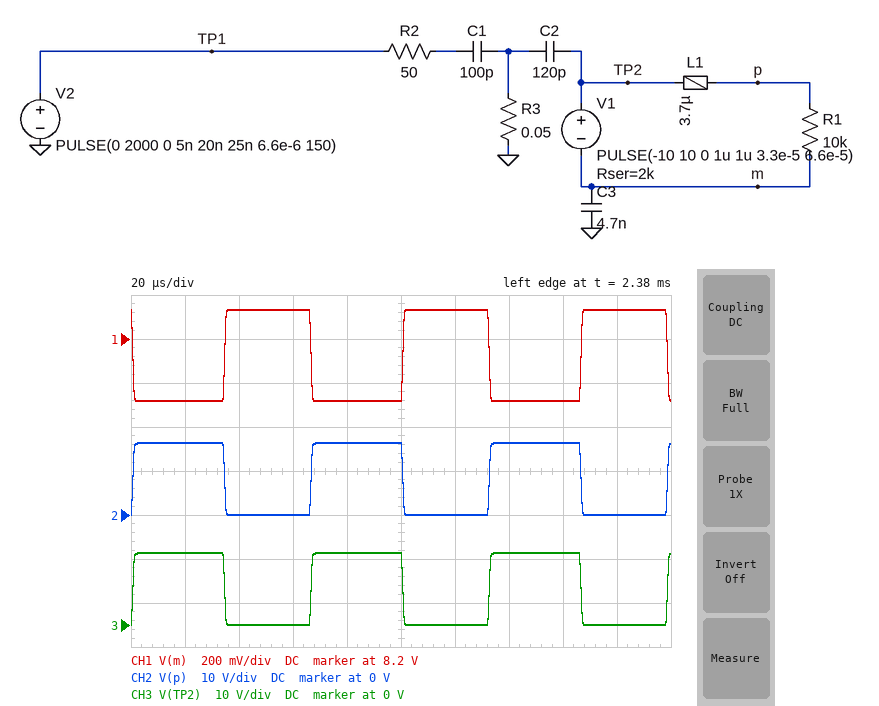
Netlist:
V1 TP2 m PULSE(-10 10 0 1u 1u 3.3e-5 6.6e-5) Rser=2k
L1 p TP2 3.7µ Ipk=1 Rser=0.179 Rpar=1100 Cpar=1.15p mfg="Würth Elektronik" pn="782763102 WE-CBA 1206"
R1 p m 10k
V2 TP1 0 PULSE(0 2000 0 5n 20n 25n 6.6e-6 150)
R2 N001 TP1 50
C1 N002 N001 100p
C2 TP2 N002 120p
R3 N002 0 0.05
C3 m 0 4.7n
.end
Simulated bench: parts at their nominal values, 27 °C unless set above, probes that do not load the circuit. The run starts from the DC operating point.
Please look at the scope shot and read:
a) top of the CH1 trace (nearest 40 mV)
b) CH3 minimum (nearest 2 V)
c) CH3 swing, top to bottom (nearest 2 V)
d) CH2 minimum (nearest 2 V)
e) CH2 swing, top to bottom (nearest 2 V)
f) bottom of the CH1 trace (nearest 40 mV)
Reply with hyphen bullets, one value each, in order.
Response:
- 8.32 V
- 0 V
- 16 V
- 0 V
- 16 V
- 7.92 V
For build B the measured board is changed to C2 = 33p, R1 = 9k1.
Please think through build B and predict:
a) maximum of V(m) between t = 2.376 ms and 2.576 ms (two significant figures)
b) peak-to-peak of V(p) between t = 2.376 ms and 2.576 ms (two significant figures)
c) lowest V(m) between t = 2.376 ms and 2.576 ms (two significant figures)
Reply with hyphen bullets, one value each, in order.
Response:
- 8.2 V
- 16 V
- 8.1 V
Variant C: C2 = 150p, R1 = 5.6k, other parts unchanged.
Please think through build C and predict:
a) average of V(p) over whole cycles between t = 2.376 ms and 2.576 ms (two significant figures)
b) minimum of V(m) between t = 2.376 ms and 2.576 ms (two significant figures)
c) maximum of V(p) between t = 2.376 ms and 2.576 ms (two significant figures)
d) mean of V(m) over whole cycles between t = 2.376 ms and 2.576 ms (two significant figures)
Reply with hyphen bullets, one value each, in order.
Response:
- 7.4 V
- 6.9 V
- 14 V
- 7.1 V
